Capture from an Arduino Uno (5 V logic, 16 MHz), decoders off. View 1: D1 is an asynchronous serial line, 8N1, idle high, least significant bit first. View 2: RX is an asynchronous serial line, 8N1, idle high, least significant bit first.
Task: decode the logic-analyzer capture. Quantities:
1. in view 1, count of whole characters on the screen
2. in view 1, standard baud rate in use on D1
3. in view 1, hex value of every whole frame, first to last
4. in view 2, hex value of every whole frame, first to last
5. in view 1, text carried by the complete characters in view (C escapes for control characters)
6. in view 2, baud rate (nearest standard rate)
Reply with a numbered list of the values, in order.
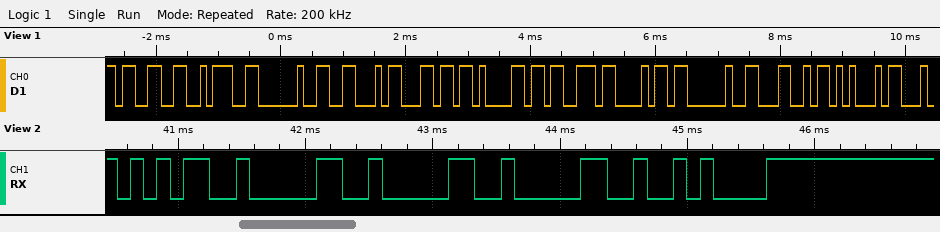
1. 11
2. 9600 baud
3. 33 3A 20 46 6C 61 73 68 20 4C 45
4. 35 30 30 30 0A
5. "3: Flash LE"
6. 9600 baud
